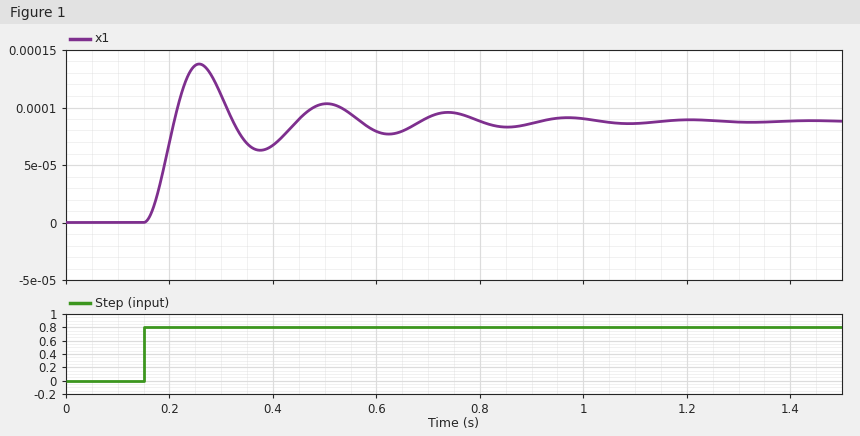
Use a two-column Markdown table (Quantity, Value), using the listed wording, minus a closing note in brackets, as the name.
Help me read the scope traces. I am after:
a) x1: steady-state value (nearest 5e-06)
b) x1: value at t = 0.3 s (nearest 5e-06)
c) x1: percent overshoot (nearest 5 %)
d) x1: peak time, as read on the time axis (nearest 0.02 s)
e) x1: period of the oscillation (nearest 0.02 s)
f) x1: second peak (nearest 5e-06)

| Quantity | Value |
|---|---|
| x1: steady-state value | 0.000090 |
| x1: value at t = 0.3 s | 0.000110 |
| x1: percent overshoot | 55 % |
| x1: peak time, as read on the time axis | 0.26 s |
| x1: period of the oscillation | 0.24 s |
| x1: second peak | 0.000105 |
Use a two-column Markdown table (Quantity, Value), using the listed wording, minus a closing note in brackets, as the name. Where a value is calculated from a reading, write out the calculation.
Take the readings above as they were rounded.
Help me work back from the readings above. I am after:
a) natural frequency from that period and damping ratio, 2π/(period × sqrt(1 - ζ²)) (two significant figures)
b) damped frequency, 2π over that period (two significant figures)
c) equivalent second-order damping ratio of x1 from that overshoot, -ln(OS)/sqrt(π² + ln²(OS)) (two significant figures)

| Quantity | Value |
|---|---|
| natural frequency from that period and damping ratio, 2π/(period × sqrt(1 - ζ²)) | 2π / (0.24 × sqrt(1 - 0.19²)) = 27 rad/s |
| damped frequency, 2π over that period | 2π / 0.24 = 26 rad/s |
| equivalent second-order damping ratio of x1 from that overshoot, -ln(OS)/sqrt(π² + ln²(OS)) | ln(0.55) = -0.598; 0.598 / sqrt(9.870 + 0.357) = 0.19 |
